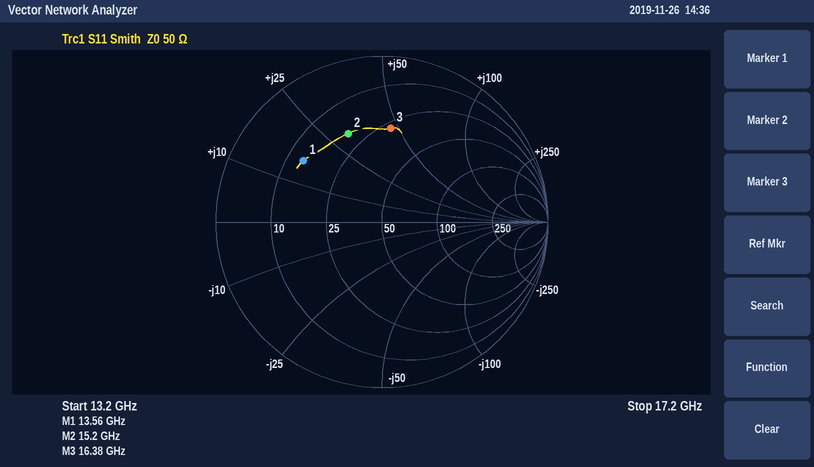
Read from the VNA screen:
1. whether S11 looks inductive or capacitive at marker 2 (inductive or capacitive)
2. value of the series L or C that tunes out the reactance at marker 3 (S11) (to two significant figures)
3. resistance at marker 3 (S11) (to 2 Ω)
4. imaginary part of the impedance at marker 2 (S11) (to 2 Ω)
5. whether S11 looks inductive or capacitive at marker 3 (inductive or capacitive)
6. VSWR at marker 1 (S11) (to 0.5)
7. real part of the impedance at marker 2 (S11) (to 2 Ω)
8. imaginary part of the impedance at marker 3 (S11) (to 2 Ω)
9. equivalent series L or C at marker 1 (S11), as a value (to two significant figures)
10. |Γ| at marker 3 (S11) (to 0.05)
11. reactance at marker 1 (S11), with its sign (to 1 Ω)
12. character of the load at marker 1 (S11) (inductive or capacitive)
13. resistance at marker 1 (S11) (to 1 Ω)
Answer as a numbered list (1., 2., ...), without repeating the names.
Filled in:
1. inductive
2. 210 fF
3. 28 Ω
4. +30 Ω
5. inductive
6. 4.0
7. 20 Ω
8. +46 Ω
9. 190 pH
10. 0.55
11. +16 Ω
12. inductive
13. 14 Ω
